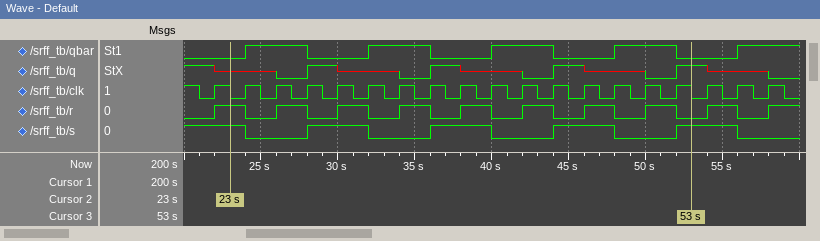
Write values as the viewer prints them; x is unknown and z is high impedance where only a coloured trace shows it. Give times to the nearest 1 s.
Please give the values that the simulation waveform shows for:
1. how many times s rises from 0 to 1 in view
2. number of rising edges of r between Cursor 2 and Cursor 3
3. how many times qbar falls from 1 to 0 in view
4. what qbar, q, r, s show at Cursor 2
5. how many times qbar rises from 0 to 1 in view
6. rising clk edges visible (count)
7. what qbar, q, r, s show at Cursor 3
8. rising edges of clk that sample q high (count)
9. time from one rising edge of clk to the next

4
7
4
qbar=0, q=x, r=1, s=1
5
19
qbar=0, q=1, r=0, s=1
5
2 s
